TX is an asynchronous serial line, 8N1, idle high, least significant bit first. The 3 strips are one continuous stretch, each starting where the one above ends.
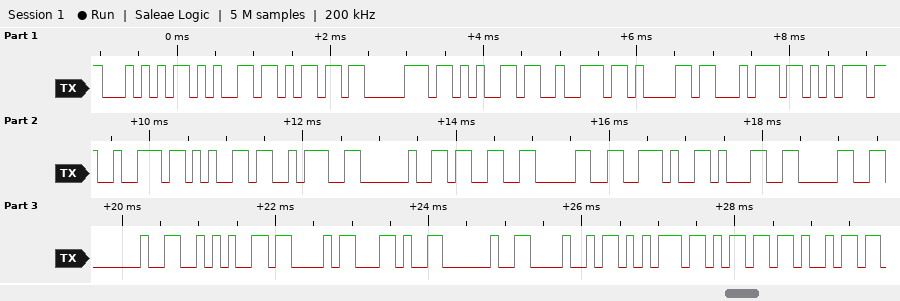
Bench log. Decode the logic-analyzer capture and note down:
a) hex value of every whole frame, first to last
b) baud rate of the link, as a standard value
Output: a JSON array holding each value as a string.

["0x54 0x65 0x6D 0x70 0x65 0x72 0x61 0x74 0x75 0x72 0x65 0x3A 0x20 0x33 0x30 0x2E 0x31 0x30 0x20 0x2A 0x43 0x2C 0x20 0x48 0x75 0x6D 0x69", "9600 baud"]
